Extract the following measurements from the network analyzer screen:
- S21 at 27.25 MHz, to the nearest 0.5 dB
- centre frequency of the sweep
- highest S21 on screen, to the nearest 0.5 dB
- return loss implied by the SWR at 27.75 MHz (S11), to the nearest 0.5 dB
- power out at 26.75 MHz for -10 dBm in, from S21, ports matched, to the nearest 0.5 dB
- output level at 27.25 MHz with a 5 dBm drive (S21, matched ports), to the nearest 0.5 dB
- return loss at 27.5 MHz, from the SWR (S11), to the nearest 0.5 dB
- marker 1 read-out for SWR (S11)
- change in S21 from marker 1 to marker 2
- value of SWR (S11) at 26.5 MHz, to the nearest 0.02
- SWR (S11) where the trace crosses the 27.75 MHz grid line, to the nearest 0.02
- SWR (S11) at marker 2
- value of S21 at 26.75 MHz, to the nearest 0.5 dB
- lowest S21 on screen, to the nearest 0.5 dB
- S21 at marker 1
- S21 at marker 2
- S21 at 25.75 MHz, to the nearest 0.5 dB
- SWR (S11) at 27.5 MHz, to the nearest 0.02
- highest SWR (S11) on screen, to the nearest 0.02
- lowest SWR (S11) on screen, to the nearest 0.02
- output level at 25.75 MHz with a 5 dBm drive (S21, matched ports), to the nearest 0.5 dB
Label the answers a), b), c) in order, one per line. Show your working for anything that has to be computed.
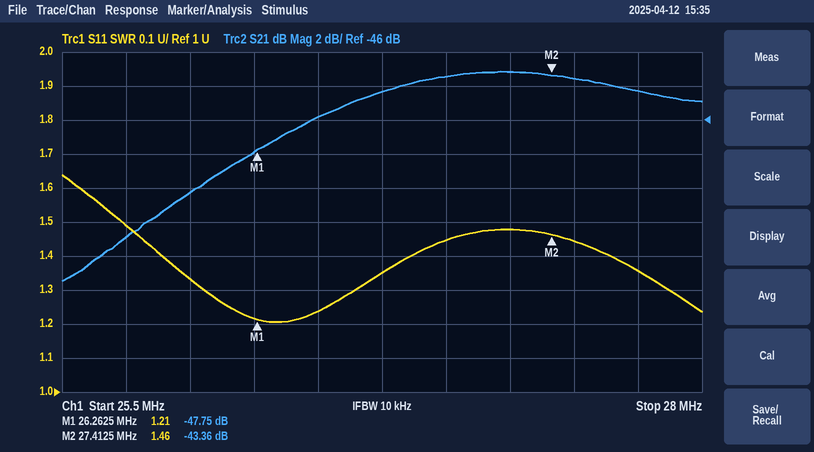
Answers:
a) -43.0 dB
b) 26.75 MHz
c) -43.0 dB
d) −20 log10((1.36 − 1)/(1.36 + 1)) ≈ 16.3 dB, so 16.5 dB to the nearest 0.5 dB
e) -10 dBm + (-44.5 dB) = -54.5 dBm
f) 5 dBm + (-43.0 dB) = -38.0 dBm
g) −20 log10((1.44 − 1)/(1.44 + 1)) ≈ 14.9 dB, so 15.0 dB to the nearest 0.5 dB
h) 1.21
i) -43.36 − (-47.75) = 4.39 dB
j) 1.24
k) 1.36
l) 1.46
m) -44.5 dB
n) -55.5 dB
o) -47.75 dB
p) -43.36 dB
q) -53.0 dB
r) 1.44
s) 1.64
t) 1.20
u) 5 dBm + (-53.0 dB) = -48.0 dBm
